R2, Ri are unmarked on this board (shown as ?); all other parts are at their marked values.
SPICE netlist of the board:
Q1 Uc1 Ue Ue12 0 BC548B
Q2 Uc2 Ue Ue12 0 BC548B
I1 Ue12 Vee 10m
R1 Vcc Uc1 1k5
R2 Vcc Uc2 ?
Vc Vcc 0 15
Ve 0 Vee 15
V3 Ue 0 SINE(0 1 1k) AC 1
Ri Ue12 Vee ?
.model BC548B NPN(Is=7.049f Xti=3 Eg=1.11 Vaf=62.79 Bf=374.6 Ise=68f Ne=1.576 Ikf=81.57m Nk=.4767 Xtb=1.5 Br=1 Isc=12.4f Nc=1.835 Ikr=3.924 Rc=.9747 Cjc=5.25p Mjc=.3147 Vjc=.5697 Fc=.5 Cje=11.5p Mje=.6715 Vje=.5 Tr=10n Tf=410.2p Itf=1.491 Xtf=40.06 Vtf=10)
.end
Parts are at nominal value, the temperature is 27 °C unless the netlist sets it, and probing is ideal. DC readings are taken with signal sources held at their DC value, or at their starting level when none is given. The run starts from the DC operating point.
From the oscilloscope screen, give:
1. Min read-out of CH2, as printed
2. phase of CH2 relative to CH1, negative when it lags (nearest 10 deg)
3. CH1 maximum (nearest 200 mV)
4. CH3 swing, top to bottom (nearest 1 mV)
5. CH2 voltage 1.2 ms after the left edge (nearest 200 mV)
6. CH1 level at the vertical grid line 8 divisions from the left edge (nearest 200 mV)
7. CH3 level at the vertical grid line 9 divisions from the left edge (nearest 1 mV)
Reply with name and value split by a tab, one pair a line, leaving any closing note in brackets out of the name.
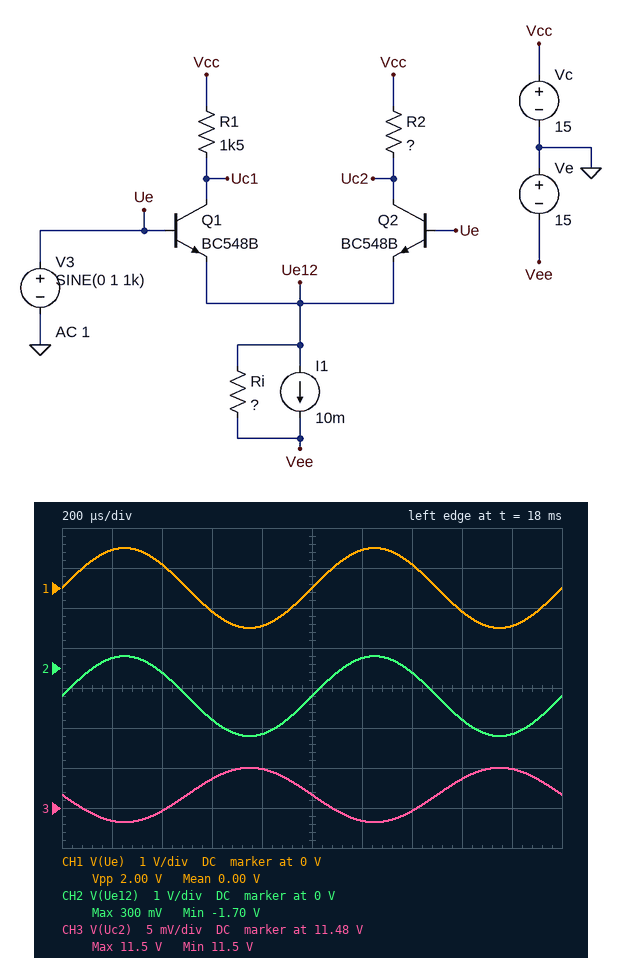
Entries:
Min read-out of CH2, as printed	-1.70 V
phase of CH2 relative to CH1, negative when it lags	0 deg
CH1 maximum	1.0 V
CH3 swing, top to bottom	7 mV
CH2 voltage 1.2 ms after the left edge	200 mV
CH1 level at the vertical grid line 8 divisions from the left edge	-600 mV
CH3 level at the vertical grid line 9 divisions from the left edge	11.490 V
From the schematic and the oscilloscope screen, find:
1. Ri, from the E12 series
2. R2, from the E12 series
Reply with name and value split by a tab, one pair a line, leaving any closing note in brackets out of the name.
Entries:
Ri, from the E12 series	150 kΩ
R2, from the E12 series	680 Ω
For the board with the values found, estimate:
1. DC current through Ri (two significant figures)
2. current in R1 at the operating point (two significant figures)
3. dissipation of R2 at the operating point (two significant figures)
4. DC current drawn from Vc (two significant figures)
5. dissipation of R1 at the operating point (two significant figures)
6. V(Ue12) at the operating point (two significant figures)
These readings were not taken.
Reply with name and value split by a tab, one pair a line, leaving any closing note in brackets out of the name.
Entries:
DC current through Ri	95 µA
current in R1 at the operating point	4.9 mA
dissipation of R2 at the operating point	18 mW
DC current drawn from Vc	10 mA
dissipation of R1 at the operating point	36 mW
V(Ue12) at the operating point	-700 mV
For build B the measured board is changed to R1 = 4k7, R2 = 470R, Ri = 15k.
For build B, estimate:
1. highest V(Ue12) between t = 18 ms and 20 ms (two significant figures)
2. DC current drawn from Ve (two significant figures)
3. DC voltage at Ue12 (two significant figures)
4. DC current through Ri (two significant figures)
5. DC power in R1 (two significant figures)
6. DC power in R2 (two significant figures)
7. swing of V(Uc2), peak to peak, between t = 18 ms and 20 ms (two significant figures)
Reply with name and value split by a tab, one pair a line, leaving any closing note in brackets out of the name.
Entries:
highest V(Ue12) between t = 18 ms and 20 ms	290 mV
DC current drawn from Ve	11 mA
DC voltage at Ue12	-710 mV
DC current through Ri	950 µA
DC power in R1	52 mW
DC power in R2	20 mW
swing of V(Uc2), peak to peak, between t = 18 ms and 20 ms	84 mV
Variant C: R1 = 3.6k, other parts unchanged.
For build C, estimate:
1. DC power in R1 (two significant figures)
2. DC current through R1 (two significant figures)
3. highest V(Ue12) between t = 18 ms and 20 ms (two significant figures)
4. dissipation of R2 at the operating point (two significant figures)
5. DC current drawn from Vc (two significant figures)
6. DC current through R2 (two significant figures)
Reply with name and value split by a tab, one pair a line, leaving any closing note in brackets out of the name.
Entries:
DC power in R1	68 mW
DC current through R1	4.3 mA
highest V(Ue12) between t = 18 ms and 20 ms	290 mV
dissipation of R2 at the operating point	21 mW
DC current drawn from Vc	9.9 mA
DC current through R2	5.6 mA
